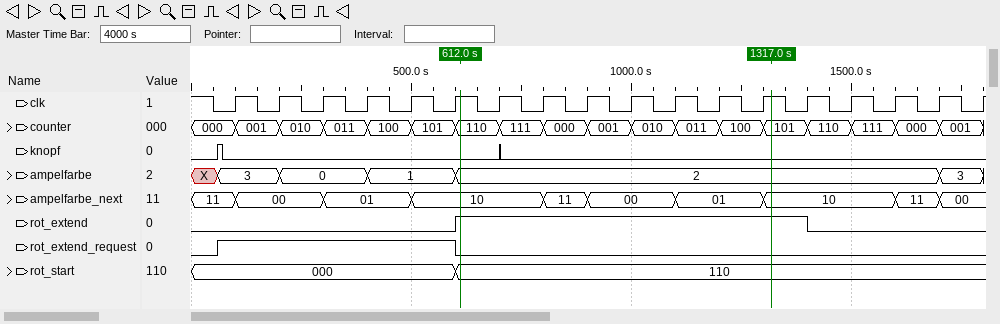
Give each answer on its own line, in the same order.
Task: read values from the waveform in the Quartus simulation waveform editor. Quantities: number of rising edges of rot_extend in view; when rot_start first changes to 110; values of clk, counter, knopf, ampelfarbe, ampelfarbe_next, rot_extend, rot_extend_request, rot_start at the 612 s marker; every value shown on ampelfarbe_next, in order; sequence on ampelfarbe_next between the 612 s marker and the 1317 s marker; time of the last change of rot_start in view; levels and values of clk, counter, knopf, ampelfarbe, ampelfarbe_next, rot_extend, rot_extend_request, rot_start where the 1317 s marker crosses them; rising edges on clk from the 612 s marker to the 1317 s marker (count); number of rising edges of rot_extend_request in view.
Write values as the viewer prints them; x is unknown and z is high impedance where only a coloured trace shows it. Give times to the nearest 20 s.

1
600 s
clk=1, counter=110, knopf=0, ampelfarbe=2, ampelfarbe_next=10, rot_extend=1, rot_extend_request=0, rot_start=110
11, 00, 01, 10, 11, 00, 01, 10, 11, 00
10, 11, 00, 01, 10
600 s
clk=1, counter=101, knopf=0, ampelfarbe=2, ampelfarbe_next=10, rot_extend=1, rot_extend_request=0, rot_start=110
7
1
